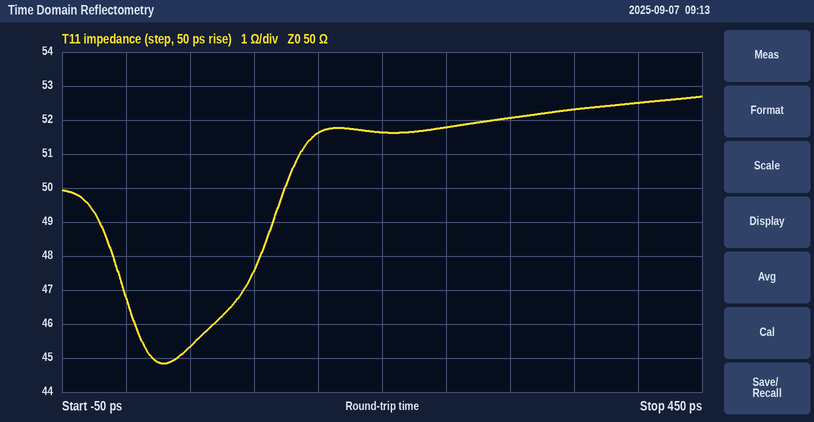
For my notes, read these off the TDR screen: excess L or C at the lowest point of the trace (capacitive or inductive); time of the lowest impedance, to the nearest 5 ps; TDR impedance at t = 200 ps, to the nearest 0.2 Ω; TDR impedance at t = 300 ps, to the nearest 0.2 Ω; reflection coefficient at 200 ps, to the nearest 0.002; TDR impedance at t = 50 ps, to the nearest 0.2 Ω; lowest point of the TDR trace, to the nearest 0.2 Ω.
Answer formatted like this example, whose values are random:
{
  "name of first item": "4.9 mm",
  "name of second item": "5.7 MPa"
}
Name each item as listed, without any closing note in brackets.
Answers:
{
  "excess L or C at the lowest point of the trace": "capacitive",
  "time of the lowest impedance, to the nearest 5 ps": "30 ps",
  "TDR impedance at t = 200 ps, to the nearest 0.2 Ω": "51.6 Ω",
  "TDR impedance at t = 300 ps, to the nearest 0.2 Ω": "52.0 Ω",
  "reflection coefficient at 200 ps, to the nearest 0.002": "+0.016",
  "TDR impedance at t = 50 ps, to the nearest 0.2 Ω": "45.4 Ω",
  "lowest point of the TDR trace, to the nearest 0.2 Ω": "44.8 Ω"
}
